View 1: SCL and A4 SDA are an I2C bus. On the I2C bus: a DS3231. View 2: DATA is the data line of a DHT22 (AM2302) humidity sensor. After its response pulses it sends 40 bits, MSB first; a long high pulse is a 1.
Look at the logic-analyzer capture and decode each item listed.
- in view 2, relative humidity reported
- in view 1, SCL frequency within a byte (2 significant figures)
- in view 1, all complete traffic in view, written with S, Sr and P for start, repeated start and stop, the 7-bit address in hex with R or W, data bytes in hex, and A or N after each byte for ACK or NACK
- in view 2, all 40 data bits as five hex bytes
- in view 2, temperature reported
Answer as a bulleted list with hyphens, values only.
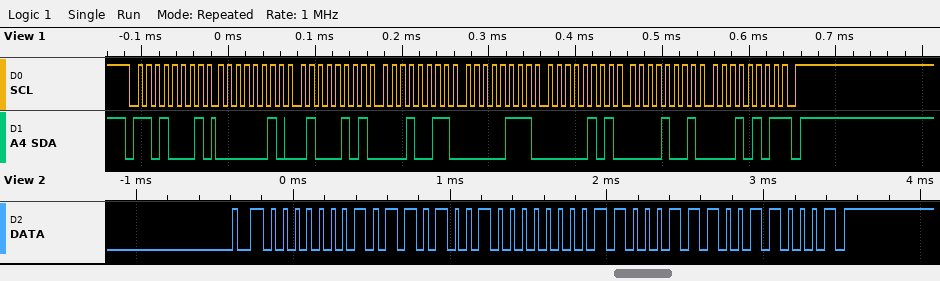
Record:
- 36.1 %
- 100 kHz
- S 68R A 02 A 45 A 13 A 07 A 05 A 09 A 15 N P
- 01 69 00 C7 31
- 19.9 °C
